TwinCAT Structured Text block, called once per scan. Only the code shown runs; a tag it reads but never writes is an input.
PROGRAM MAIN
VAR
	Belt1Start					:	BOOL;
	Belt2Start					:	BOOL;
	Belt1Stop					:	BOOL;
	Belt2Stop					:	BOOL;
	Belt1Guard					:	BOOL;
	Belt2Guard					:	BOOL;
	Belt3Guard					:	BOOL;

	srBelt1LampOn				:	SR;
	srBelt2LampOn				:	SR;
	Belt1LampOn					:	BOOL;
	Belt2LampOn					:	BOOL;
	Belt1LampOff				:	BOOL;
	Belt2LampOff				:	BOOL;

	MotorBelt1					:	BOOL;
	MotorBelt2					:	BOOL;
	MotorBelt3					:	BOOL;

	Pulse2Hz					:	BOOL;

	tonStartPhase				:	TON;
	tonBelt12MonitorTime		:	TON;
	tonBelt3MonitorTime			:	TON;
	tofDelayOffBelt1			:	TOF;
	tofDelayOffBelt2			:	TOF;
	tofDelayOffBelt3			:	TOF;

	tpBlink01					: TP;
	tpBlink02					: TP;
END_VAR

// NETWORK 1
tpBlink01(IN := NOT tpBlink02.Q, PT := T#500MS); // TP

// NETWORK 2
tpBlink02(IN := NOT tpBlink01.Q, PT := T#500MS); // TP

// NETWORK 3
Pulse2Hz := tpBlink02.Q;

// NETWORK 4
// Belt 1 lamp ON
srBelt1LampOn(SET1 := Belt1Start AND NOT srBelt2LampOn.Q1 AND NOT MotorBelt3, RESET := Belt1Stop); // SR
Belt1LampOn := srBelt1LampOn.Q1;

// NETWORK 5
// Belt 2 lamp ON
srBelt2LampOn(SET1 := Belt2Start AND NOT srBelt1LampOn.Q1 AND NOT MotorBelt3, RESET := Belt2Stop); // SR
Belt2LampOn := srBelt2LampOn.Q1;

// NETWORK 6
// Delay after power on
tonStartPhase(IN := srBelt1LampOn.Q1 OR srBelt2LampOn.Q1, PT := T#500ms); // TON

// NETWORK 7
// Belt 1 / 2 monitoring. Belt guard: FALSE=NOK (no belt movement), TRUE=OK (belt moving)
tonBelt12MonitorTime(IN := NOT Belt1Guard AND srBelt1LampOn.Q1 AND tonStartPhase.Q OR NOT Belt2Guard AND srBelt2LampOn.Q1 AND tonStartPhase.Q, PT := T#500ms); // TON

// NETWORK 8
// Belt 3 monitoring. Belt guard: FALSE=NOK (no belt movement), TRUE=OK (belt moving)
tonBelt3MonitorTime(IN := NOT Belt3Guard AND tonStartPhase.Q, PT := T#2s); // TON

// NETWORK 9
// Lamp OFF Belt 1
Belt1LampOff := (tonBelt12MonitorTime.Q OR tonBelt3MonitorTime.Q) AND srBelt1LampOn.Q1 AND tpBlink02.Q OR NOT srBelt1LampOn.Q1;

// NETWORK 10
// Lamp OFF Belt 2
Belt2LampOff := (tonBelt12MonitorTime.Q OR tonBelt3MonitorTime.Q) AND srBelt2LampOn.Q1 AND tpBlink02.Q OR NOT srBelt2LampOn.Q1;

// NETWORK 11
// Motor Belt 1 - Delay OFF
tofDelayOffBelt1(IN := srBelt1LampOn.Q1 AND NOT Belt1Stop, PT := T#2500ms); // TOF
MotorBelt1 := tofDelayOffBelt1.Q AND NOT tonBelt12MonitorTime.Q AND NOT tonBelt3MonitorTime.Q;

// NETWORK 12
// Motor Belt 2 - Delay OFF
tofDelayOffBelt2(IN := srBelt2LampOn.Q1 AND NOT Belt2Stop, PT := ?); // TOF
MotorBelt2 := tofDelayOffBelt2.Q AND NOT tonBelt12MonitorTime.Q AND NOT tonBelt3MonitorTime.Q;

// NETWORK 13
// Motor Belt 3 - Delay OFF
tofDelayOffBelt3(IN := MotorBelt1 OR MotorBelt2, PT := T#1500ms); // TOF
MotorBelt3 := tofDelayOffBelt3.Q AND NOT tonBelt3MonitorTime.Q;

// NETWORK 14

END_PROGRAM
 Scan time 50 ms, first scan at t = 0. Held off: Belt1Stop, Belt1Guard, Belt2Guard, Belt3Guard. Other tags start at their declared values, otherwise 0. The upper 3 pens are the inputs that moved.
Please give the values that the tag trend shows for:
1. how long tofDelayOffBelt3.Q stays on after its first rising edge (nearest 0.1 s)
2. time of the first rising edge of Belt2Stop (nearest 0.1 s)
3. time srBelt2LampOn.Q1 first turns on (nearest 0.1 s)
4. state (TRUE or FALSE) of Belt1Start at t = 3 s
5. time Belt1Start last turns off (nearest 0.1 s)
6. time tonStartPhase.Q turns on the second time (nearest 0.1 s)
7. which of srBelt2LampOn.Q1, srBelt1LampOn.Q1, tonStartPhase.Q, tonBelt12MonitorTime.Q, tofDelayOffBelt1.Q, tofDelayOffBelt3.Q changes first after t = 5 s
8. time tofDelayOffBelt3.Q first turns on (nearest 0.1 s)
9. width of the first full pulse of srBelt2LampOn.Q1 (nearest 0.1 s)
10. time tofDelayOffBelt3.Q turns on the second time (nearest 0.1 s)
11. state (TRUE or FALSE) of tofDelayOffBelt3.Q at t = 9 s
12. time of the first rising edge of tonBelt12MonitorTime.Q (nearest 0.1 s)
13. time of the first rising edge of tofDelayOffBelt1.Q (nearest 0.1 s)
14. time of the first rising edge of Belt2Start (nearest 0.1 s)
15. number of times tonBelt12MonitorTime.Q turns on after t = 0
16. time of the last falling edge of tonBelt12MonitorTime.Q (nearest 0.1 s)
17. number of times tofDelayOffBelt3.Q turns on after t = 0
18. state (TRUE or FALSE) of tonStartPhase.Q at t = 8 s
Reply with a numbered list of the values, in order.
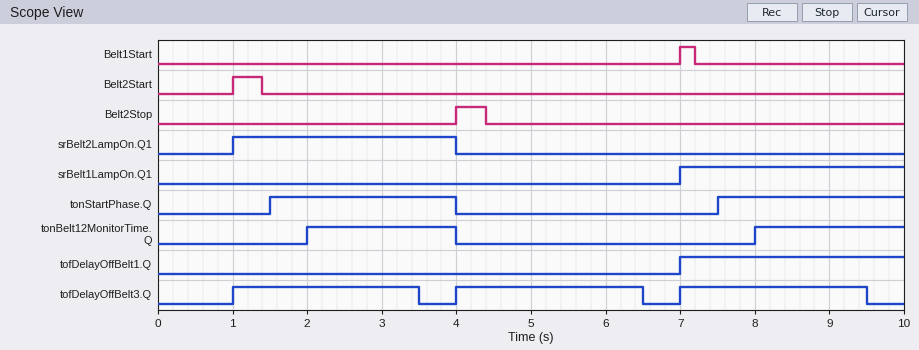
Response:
1. 2.5 s
2. 4.0 s
3. 1.0 s
4. FALSE
5. 7.2 s
6. 7.5 s
7. tofDelayOffBelt3.Q
8. 1.0 s
9. 3.0 s
10. 4.0 s
11. TRUE
12. 2.0 s
13. 7.0 s
14. 1.0 s
15. 2
16. 4.0 s
17. 3
18. TRUE
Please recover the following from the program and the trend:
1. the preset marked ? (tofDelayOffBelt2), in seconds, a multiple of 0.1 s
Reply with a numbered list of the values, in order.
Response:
1. 1.0 s
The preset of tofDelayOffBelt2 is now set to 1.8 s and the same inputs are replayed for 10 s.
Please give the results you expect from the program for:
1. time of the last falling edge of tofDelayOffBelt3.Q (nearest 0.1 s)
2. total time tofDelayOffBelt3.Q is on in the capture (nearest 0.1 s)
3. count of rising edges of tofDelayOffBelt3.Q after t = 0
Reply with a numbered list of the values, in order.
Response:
1. 7.3 s
2. 5.8 s
3. 2
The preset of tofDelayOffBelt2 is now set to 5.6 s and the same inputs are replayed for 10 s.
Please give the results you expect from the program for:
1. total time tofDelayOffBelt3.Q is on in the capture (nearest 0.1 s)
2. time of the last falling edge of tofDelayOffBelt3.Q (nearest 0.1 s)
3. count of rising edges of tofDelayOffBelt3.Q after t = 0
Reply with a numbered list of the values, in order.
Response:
1. 8.5 s
2. 3.5 s
3. 2
